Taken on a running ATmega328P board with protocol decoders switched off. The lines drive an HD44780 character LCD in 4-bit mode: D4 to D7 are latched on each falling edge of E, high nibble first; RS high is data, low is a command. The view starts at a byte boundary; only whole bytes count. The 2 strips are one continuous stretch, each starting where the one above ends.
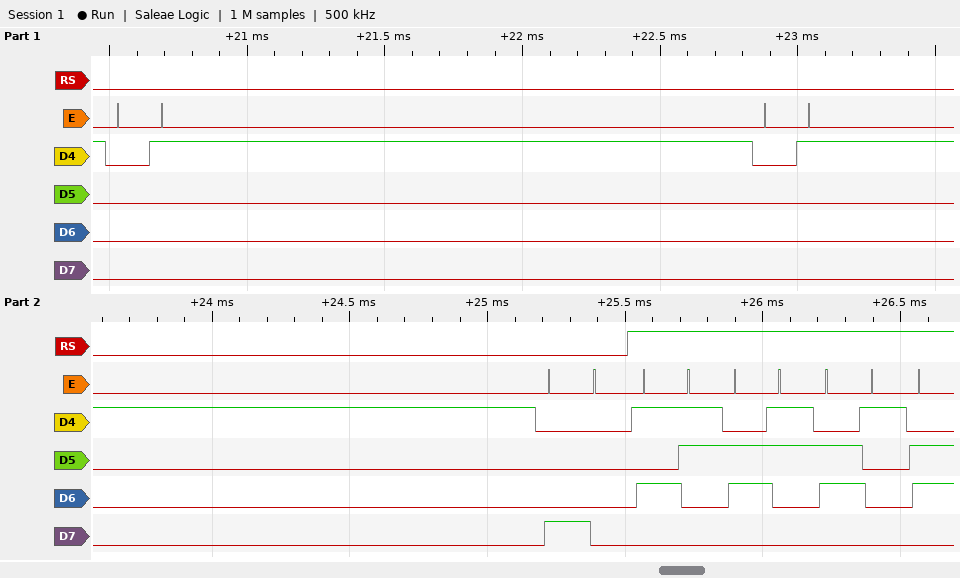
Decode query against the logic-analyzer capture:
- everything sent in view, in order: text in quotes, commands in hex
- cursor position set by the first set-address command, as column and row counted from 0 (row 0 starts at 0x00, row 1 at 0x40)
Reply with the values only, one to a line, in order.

0x01 0x01 0x80 "Sca"
column 0, row 0
